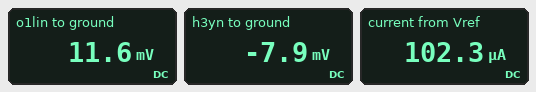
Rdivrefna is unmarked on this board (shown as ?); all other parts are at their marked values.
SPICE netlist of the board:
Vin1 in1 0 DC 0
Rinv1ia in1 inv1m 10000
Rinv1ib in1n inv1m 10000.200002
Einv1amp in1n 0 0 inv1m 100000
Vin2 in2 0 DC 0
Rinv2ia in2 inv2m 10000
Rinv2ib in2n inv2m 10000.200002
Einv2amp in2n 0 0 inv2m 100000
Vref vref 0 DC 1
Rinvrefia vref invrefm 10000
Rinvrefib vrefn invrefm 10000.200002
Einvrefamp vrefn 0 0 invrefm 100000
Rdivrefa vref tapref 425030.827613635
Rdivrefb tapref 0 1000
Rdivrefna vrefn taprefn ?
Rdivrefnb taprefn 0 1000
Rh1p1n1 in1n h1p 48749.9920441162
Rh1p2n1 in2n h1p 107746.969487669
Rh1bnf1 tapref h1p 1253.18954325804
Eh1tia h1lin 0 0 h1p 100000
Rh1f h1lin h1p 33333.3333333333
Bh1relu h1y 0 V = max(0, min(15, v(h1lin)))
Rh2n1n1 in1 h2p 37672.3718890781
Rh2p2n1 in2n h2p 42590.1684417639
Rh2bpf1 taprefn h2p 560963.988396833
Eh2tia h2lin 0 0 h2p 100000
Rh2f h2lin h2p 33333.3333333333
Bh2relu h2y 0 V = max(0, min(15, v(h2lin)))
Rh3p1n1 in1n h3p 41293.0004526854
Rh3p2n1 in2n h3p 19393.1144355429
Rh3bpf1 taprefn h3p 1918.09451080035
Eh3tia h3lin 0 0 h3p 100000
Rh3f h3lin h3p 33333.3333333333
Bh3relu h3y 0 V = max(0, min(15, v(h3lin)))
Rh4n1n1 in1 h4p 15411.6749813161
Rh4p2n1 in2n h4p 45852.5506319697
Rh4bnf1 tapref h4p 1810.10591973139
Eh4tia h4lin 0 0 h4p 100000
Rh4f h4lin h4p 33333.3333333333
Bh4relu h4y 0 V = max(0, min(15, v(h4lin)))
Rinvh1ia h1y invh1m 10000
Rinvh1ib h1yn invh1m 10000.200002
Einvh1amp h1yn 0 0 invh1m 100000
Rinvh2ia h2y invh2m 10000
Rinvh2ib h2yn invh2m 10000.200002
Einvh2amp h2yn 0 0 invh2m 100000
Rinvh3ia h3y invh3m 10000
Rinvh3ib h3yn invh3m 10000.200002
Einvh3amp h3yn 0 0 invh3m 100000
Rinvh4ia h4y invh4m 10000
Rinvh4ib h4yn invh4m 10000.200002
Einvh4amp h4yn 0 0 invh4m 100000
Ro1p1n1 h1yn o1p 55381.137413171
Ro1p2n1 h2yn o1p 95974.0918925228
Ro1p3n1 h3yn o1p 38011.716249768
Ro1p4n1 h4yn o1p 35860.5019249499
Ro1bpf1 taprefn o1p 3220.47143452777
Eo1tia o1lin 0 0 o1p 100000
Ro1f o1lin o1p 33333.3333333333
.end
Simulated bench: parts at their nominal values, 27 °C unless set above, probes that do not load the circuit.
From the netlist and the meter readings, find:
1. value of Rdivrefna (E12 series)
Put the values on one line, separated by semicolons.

1.2 MΩ
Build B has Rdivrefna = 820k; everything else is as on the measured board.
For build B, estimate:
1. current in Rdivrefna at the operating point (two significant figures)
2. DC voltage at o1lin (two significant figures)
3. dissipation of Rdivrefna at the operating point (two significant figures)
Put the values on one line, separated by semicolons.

1.2 µA; 17 mV; 1.2 µW
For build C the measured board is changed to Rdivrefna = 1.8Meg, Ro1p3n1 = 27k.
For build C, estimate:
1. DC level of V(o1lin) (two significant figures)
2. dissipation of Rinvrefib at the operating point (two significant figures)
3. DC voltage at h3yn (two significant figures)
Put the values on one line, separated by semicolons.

9.6 mV; 100 µW; -5.3 mV
